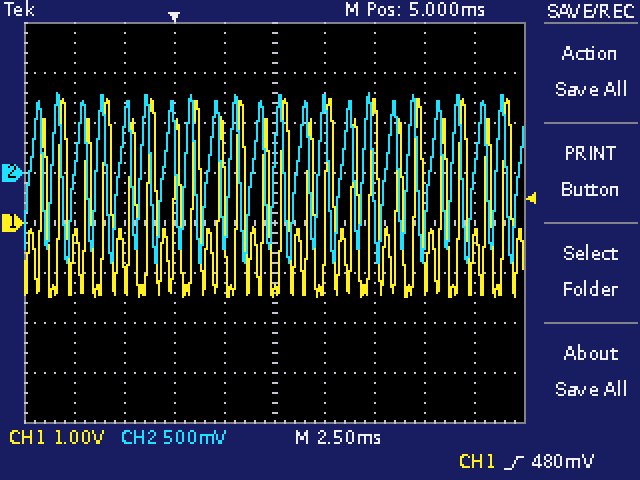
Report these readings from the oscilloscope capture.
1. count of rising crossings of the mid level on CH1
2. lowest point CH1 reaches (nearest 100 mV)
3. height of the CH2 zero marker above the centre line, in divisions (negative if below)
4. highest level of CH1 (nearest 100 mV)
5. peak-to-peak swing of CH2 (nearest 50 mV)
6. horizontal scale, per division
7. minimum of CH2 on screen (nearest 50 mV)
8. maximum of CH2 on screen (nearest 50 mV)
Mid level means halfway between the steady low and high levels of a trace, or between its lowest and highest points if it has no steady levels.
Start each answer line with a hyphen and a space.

- 22
- -1.5 V
- +1.0 div
- 2.5 V
- 1.70 V
- 2.5 ms
- -900 mV
- 800 mV
